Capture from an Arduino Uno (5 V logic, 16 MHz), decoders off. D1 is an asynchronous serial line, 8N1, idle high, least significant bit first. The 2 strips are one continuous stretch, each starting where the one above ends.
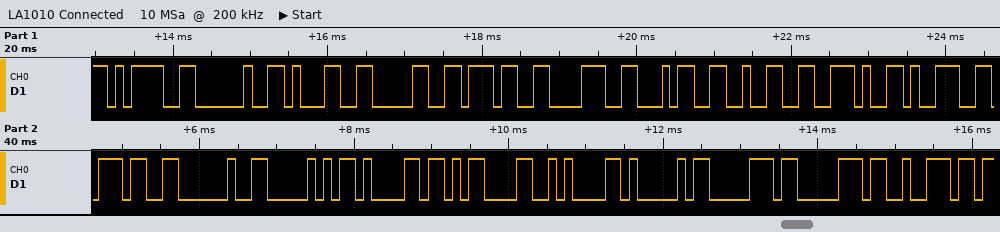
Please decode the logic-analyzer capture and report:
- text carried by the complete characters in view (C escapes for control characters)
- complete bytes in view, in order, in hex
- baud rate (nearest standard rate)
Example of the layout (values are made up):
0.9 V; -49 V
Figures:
"= 107842.97 Pa\r\nAppr"; 3D 20 31 30 37 38 34 32 2E 39 37 20 50 61 0D 0A 41 70 70 72; 9600 baud
